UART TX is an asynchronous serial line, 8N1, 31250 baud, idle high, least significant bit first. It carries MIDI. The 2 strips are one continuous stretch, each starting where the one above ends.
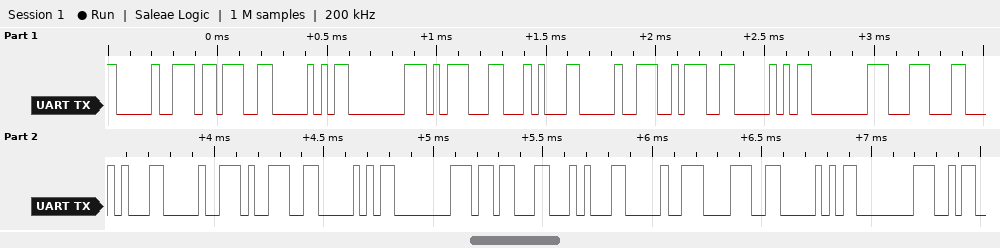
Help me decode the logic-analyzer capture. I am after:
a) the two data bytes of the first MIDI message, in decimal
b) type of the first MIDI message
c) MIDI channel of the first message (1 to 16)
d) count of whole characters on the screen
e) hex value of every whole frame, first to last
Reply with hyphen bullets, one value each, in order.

- 59, 80
- Note On
- 1
- 22
- 90 3B 50 80 1D 14 90 3A 50 80 1C 14 90 39 50 80 1B 14 90 38 50 80
